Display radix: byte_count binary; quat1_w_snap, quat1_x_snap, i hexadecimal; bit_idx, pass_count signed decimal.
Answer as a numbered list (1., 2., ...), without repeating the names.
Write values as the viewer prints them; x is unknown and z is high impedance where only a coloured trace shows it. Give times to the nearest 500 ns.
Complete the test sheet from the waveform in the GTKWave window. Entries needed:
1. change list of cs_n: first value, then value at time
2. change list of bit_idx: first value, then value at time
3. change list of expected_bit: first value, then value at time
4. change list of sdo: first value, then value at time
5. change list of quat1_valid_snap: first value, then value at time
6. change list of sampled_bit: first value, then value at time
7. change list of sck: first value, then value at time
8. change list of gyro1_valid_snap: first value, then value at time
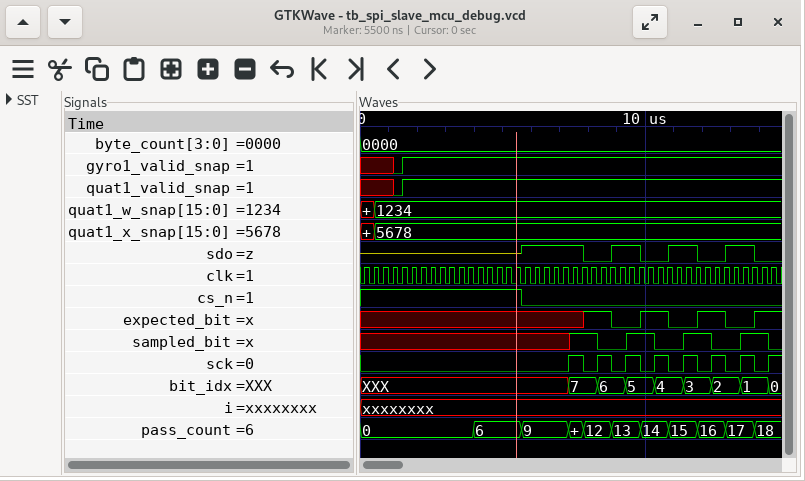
1. 1, 0 at 5500 ns
2. XXX, 7 at 7500 ns, 6 at 8500 ns, 5 at 9500 ns, 4 at 10500 ns, 3 at 11500 ns, 2 at 12500 ns, 1 at 13500 ns, 0 at 14500 ns
3. x, 1 at 8000 ns, 0 at 9000 ns, 1 at 10000 ns, 0 at 11000 ns, 1 at 12000 ns, 0 at 13000 ns, 1 at 14000 ns
4. z, 1 at 5500 ns, 0 at 8000 ns, 1 at 9000 ns, 0 at 10000 ns, 1 at 11000 ns, 0 at 12000 ns, 1 at 13000 ns, 0 at 14000 ns
5. x, 0 at 1000 ns, 1 at 1500 ns
6. x, 1 at 7500 ns, 0 at 8500 ns, 1 at 9500 ns, 0 at 10500 ns, 1 at 11500 ns, 0 at 12500 ns, 1 at 13500 ns, 0 at 14500 ns
7. 0, 1 at 7500 ns, 0 at 8000 ns, 1 at 8500 ns, 0 at 9000 ns, 1 at 9500 ns, 0 at 10000 ns, 1 at 10500 ns, 0 at 11000 ns, 1 at 11500 ns, 0 at 12000 ns, 1 at 12500 ns, 0 at 13000 ns, 1 at 13500 ns, 0 at 14000 ns, 1 at 14500 ns
8. x, 0 at 1000 ns, 1 at 1500 ns
